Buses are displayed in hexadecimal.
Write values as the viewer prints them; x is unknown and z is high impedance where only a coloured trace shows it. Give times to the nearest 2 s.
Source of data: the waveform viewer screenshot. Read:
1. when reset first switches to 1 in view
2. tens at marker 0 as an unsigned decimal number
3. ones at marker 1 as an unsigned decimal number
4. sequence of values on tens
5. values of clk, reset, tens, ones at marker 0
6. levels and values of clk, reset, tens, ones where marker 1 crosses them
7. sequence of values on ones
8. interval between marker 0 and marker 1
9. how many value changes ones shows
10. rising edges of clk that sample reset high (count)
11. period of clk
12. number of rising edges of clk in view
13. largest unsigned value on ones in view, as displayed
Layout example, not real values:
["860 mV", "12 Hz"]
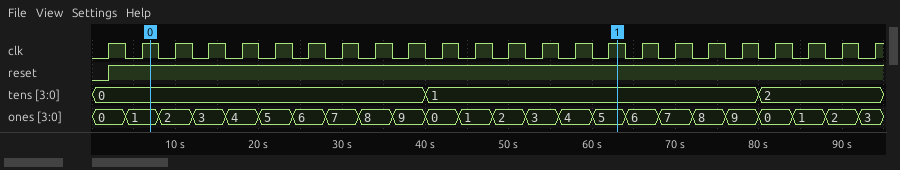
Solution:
["2 s", "0", "5", "0, 1, 2", "clk=1, reset=1, tens=0, ones=1", "clk=1, reset=1, tens=1, ones=5", "0, 1, 2, 3, 4, 5, 6, 7, 8, 9, 0, 1, 2, 3, 4, 5, 6, 7, 8, 9, 0, 1, 2, 3", "56 s", "23", "23", "4 s", "24", "9"]
